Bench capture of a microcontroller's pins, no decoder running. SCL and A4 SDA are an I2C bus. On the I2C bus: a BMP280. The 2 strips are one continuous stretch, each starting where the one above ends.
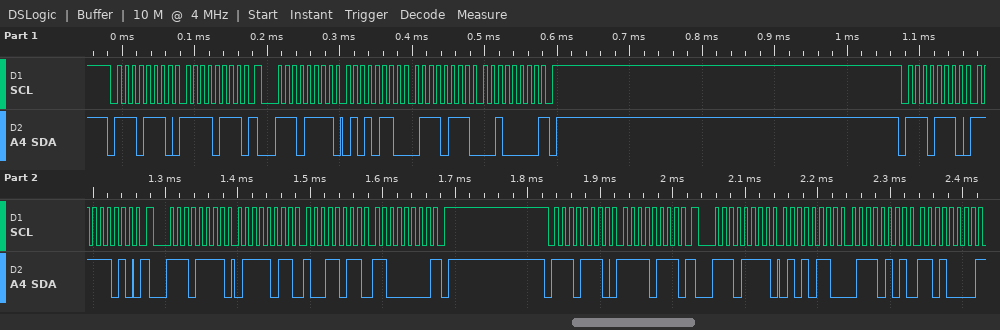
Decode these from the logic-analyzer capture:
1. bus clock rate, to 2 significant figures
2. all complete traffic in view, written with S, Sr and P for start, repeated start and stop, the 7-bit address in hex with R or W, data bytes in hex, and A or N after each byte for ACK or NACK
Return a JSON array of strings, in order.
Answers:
["100 kHz", "S 77W A F7 A Sr 77R A 56 A 77 A 20 N P S 77W A FA A Sr 77R A 7B A 9B A C0 N P S 77W A F7 A Sr 77R A 56 A 75 A D0 N"]
